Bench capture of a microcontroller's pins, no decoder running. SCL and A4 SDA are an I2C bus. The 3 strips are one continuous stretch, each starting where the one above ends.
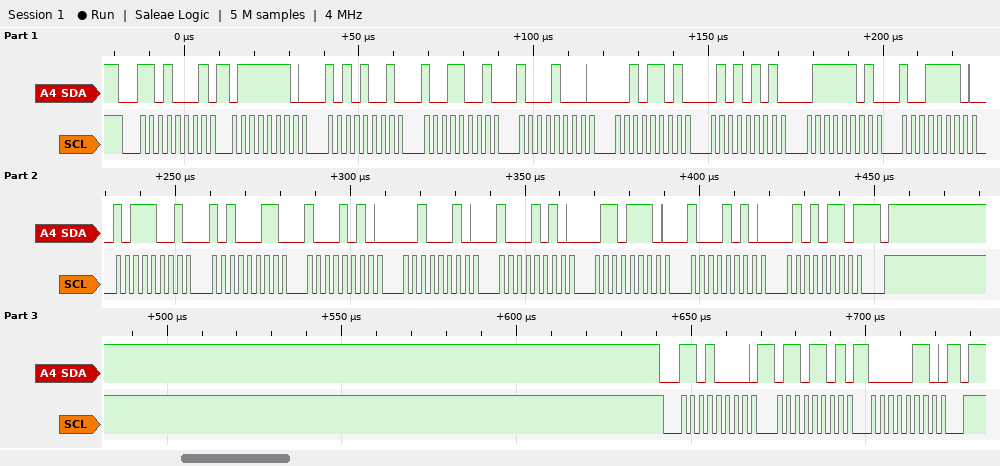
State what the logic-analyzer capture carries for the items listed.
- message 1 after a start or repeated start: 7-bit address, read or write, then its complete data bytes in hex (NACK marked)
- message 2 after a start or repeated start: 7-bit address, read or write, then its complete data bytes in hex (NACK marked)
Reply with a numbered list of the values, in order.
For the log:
1. 0x68 read: 7E A9 99 88 2D 55 7D 9E B9 A3 8A 22 8A 6E 8A 56 NACK
2. 0x68 write: 6D 06
